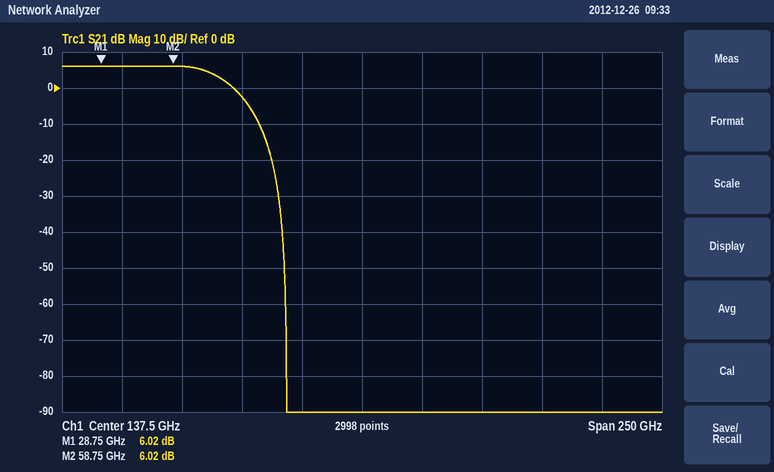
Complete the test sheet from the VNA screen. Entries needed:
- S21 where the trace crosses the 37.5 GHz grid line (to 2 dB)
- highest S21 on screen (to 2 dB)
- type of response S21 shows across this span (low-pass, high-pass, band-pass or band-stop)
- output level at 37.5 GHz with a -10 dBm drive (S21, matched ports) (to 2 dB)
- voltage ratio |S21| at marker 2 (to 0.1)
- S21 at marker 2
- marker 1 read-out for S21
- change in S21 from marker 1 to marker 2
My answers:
6 dB
6 dB
low-pass
-4 dBm
2.0
6.02 dB
6.02 dB
0.00 dB
